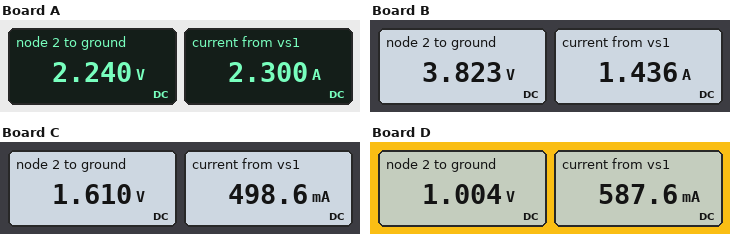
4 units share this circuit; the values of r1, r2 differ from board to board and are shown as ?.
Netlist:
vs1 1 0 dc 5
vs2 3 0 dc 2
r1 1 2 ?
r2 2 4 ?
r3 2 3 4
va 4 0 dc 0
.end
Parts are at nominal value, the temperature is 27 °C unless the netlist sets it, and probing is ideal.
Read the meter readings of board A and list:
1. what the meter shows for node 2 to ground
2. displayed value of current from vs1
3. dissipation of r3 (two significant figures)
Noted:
2.240 V
2.300 A
14 mW
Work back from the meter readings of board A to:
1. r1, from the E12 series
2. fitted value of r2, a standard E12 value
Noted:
1.2 Ω
1 Ω
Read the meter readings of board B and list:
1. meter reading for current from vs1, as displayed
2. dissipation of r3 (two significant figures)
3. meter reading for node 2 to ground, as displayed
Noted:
1.436 A
830 mW
3.823 V
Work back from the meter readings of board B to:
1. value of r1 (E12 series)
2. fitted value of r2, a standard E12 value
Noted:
0.82 Ω
3.9 Ω
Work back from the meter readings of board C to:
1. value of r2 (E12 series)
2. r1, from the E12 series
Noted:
2.7 Ω
6.8 Ω
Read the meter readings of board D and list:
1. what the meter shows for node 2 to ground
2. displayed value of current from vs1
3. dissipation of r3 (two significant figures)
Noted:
1.004 V
587.6 mA
250 mW
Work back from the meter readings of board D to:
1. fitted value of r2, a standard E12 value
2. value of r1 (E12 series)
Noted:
1.2 Ω
6.8 Ω
